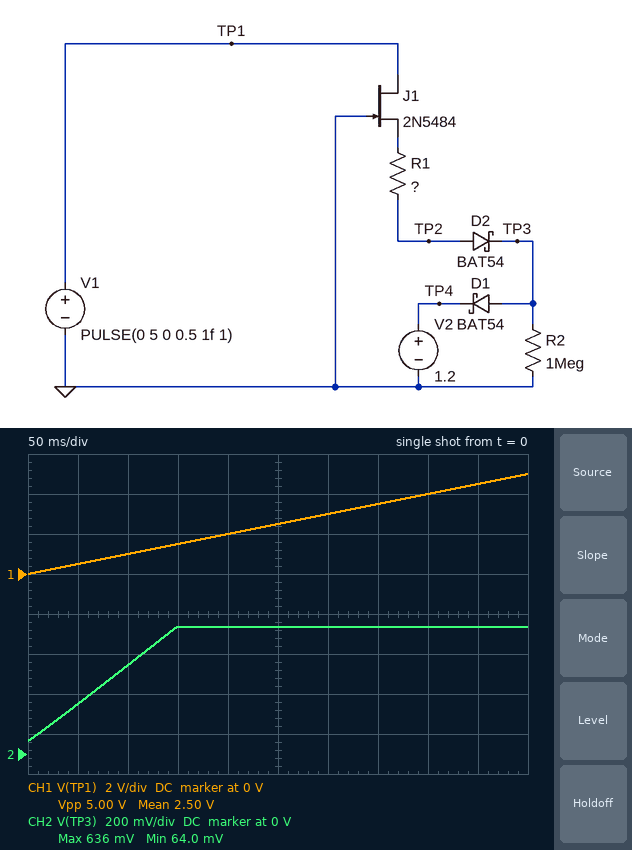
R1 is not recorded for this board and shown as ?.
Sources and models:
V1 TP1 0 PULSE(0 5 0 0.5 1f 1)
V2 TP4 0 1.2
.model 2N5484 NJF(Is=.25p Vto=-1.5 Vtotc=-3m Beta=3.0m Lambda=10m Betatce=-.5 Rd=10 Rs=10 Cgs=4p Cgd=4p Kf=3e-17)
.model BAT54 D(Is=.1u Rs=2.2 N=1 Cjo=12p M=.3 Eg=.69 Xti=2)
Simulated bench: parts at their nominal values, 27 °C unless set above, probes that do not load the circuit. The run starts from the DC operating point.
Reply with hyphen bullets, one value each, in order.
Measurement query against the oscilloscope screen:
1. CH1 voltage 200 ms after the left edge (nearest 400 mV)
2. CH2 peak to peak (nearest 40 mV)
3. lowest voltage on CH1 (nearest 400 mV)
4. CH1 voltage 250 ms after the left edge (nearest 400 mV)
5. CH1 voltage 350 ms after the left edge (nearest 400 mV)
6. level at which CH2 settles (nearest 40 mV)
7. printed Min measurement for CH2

- 2.0 V
- 560 mV
- 0 V
- 2.4 V
- 3.6 V
- 640 mV
- 64.0 mV
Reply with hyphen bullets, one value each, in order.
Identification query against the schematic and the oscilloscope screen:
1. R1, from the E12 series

- 1.5 MΩ
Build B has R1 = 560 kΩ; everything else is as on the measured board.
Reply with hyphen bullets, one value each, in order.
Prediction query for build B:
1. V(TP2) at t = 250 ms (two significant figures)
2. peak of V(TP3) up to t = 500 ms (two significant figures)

- 1.0 V
- 950 mV
